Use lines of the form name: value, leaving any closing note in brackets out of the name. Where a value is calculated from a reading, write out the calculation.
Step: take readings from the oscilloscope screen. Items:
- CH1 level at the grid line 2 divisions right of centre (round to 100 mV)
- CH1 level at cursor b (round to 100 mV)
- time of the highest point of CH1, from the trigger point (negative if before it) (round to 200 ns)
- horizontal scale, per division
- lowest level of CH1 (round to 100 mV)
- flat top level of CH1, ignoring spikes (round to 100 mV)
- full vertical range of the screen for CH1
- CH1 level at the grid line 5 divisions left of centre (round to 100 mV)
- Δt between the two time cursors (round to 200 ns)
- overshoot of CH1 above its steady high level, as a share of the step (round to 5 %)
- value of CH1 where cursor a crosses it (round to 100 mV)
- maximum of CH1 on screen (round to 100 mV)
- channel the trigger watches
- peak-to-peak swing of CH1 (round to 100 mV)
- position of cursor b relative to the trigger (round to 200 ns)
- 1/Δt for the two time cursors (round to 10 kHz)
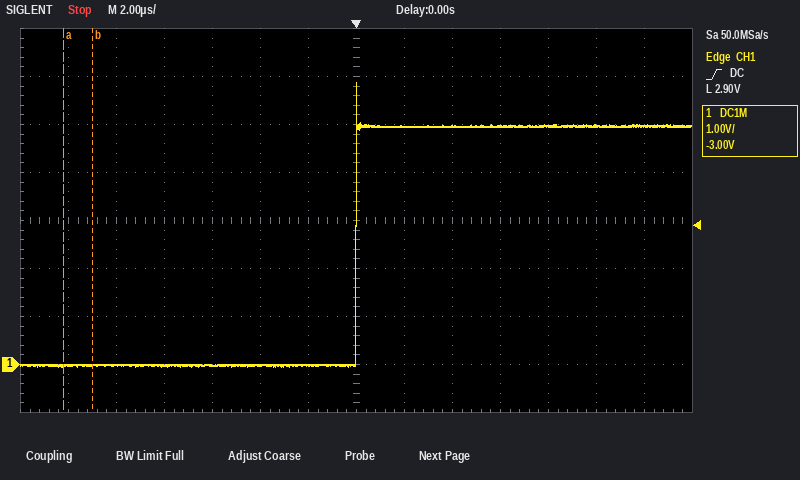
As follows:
CH1 level at the grid line 2 divisions right of centre: 5.0 V
CH1 level at cursor b: 0.0 V
time of the highest point of CH1, from the trigger point (negative if before it): 0.0 µs
horizontal scale, per division: 2 µs
lowest level of CH1: 0.0 V
flat top level of CH1, ignoring spikes: 5.0 V
full vertical range of the screen for CH1: 8 V
CH1 level at the grid line 5 divisions left of centre: 0.0 V
Δt between the two time cursors: 1.2 µs
overshoot of CH1 above its steady high level, as a share of the step: 20 %
value of CH1 where cursor a crosses it: 0.0 V
maximum of CH1 on screen: 5.9 V
channel the trigger watches: CH1
peak-to-peak swing of CH1: 5.9 V − (0.0 V) = 5.9 V
position of cursor b relative to the trigger: -11.0 µs
1/Δt for the two time cursors: 1 / 1.2 µs ≈ 830 kHz
